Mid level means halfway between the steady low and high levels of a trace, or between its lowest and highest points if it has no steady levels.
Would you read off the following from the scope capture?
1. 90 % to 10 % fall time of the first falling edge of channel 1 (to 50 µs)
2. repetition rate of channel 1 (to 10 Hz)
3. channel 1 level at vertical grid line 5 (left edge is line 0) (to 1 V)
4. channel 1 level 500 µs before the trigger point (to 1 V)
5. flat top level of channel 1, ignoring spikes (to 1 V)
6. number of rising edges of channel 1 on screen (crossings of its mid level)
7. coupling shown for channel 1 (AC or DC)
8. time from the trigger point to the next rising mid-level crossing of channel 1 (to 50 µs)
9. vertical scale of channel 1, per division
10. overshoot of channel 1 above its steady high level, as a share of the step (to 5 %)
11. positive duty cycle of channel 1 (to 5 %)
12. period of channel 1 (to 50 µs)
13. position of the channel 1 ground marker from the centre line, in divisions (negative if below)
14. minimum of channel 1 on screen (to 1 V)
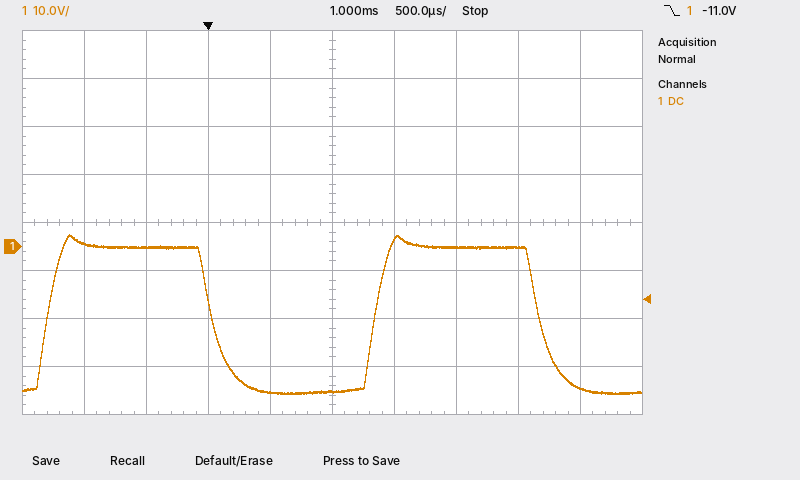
300 µs
380 Hz
-30 V
0 V
0 V
2
DC
1.35 ms
10 V
10 %
50 %
2.65 ms
-0.5 div
-31 V
